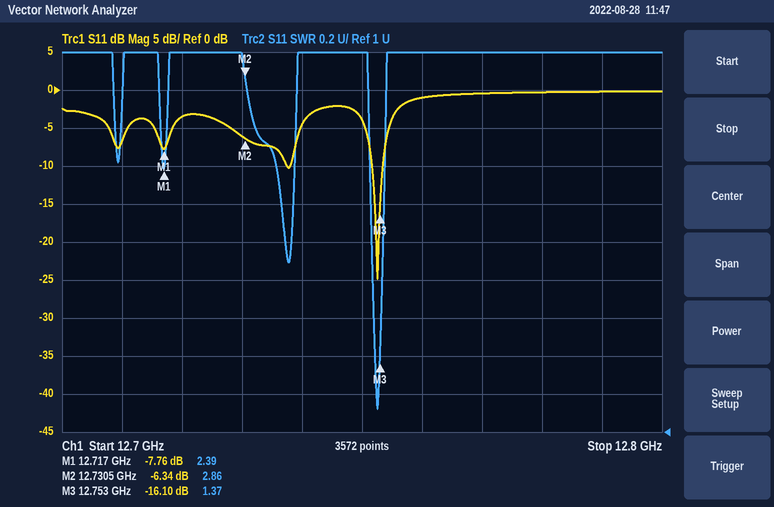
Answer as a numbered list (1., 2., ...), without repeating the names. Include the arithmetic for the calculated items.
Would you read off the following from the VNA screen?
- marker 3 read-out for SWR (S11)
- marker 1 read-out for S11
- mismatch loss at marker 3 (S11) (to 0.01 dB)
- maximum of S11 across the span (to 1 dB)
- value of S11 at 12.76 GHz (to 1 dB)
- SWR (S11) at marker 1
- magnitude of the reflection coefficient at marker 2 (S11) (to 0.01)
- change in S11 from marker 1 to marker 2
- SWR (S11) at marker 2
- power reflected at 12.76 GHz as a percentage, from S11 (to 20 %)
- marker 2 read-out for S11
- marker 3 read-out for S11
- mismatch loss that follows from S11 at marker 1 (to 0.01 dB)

1. 1.37
2. -7.76 dB
3. −10 log10(1 − 10^(-16.1/10)) ≈ 0.11 dB
4. 0 dB
5. -1 dB
6. 2.39
7. 10^(-6.34/20) ≈ 0.48
8. -6.34 − (-7.76) = 1.42 dB
9. 2.86
10. 10^(-1/10) ≈ 79.4 %, so 80 % to the nearest 20 %
11. -6.34 dB
12. -16.10 dB
13. −10 log10(1 − 10^(-7.76/10)) ≈ 0.80 dB
